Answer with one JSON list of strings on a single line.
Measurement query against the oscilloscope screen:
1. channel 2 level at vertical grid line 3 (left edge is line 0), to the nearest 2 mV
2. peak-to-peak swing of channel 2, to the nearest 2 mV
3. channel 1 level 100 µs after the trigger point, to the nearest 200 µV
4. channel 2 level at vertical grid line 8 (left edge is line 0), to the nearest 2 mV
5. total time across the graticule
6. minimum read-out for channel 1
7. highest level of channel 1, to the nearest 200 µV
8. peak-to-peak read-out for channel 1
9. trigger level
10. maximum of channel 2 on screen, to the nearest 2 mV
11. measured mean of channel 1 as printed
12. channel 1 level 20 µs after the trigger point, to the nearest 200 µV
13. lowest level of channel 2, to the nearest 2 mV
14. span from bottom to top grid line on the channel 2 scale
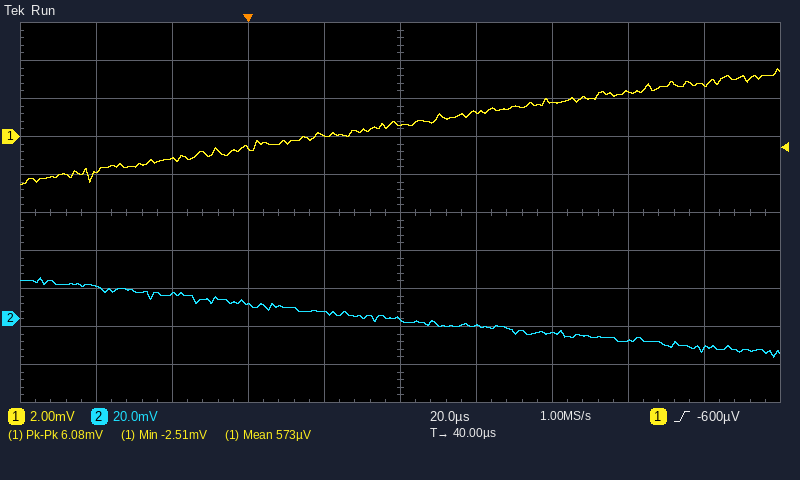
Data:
["8 mV", "42 mV", "2.4 mV", "-12 mV", "200 µs", "-2.51 mV", "3.6 mV", "6.08 mV", "-600 µV", "22 mV", "573 µV", "0.0 mV", "-20 mV", "200 mV"]
